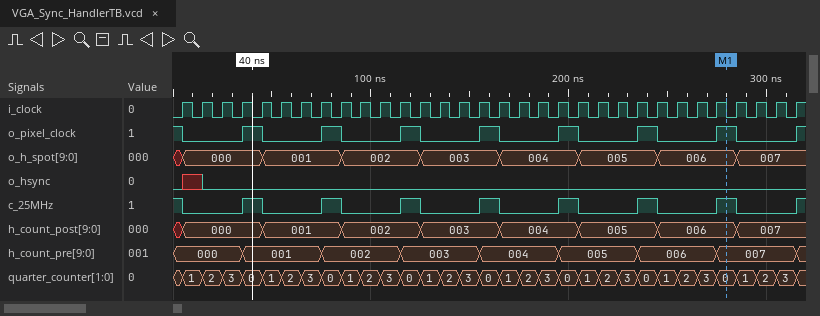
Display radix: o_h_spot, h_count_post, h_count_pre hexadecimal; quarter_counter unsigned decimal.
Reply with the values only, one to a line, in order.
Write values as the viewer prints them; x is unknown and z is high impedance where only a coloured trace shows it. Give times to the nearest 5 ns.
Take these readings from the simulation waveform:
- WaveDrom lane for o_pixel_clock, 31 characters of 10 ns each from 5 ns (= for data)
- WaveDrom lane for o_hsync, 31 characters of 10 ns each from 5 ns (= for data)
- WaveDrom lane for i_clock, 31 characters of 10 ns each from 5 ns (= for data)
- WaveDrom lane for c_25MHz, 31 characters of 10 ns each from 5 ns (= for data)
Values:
{name: 'o_pixel_clock', wave: '0..10..10..10..10..10..10..10..'}
{name: 'o_hsync', wave: 'x0.............................'}
{name: 'i_clock', wave: 'p..............................'}
{name: 'c_25MHz', wave: '0..10..10..10..10..10..10..10..'}
